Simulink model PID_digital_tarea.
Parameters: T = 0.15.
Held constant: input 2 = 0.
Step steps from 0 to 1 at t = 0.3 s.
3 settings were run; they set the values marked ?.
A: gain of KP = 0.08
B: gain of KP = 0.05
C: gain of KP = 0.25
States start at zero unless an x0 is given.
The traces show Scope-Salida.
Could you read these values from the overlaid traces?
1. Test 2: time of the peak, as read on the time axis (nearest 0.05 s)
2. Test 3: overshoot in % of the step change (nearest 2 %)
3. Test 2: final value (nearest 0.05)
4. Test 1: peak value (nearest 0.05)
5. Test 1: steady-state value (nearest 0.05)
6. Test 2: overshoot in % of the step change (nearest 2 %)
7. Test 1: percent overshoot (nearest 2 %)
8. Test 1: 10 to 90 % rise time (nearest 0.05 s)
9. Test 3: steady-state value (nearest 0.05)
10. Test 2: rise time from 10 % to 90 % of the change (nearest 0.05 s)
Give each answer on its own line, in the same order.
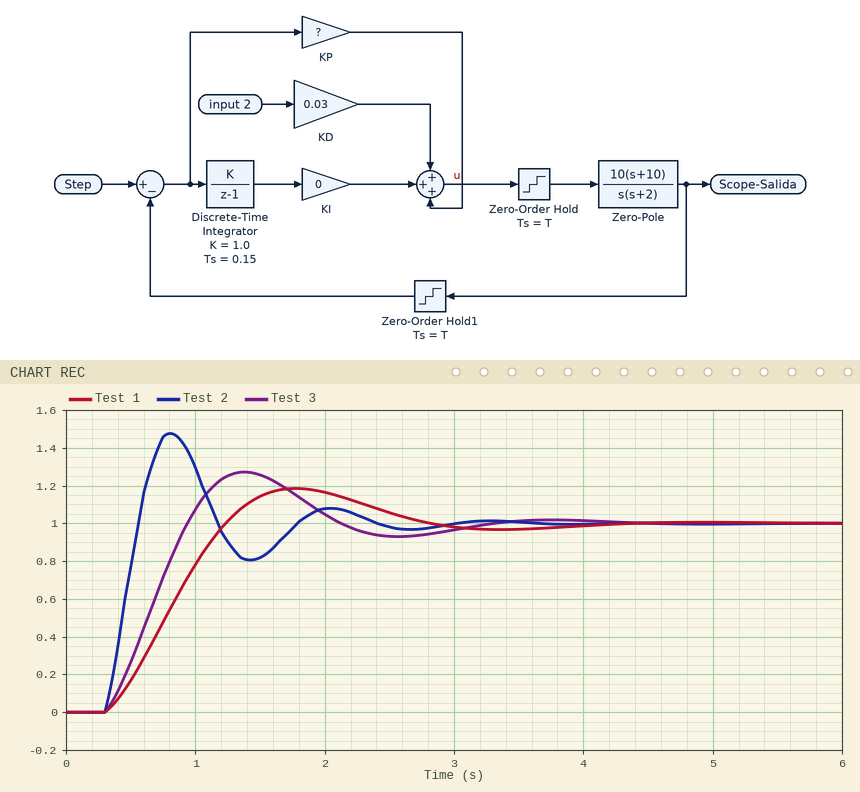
0.80 s
28 %
1.00
1.20
1.00
48 %
18 %
0.70 s
1.00
0.20 s
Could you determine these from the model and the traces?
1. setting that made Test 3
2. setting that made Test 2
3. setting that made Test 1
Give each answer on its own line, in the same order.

A
C
B
